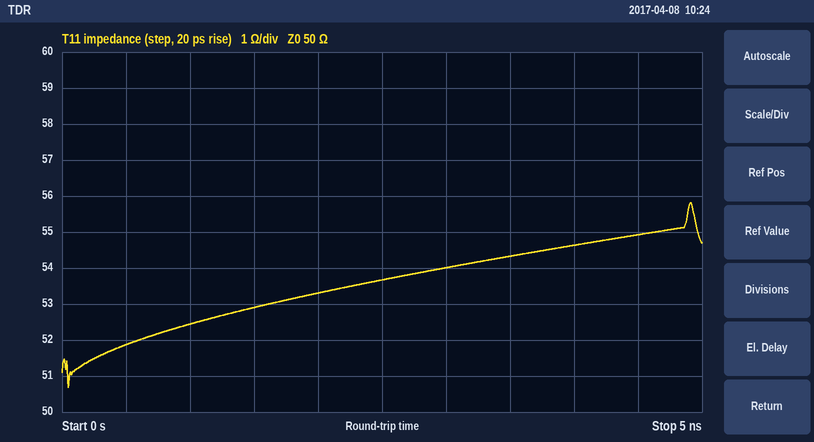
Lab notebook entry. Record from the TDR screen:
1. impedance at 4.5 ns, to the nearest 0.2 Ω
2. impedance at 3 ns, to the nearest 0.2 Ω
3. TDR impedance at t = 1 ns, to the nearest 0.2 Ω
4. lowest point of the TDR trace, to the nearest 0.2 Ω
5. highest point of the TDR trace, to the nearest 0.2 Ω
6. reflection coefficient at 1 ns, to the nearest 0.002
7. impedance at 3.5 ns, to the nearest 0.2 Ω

55.0 Ω
54.0 Ω
52.4 Ω
50.6 Ω
55.8 Ω
+0.024
54.4 Ω
